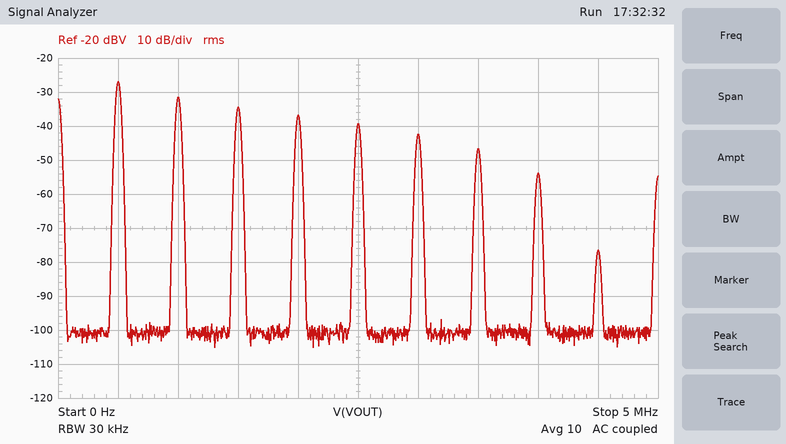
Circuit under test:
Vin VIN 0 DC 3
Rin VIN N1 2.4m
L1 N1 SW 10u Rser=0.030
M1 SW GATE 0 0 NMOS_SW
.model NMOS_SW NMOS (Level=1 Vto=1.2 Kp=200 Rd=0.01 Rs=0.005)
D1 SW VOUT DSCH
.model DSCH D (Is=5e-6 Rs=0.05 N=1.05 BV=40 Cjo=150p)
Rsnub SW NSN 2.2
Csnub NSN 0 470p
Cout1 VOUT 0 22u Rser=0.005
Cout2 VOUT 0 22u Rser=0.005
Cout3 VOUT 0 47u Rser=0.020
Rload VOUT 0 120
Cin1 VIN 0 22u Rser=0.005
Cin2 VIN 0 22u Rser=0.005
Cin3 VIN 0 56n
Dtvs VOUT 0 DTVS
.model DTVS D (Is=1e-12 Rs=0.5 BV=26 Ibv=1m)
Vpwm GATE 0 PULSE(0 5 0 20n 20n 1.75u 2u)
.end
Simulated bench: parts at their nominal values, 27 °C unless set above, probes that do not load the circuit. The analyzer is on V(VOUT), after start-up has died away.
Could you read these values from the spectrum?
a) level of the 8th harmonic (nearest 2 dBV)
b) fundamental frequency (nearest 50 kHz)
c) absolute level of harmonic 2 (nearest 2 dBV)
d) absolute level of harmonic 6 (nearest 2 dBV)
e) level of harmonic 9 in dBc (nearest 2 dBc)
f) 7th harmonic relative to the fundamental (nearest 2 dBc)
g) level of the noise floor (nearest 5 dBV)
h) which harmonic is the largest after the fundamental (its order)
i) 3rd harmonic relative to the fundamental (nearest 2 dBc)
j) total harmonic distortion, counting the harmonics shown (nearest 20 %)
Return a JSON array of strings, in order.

["-54 dBV", "500 kHz", "-32 dBV", "-42 dBV", "-50 dBc", "-20 dBc", "-100 dBV", "2", "-8 dBc", "80 %"]
